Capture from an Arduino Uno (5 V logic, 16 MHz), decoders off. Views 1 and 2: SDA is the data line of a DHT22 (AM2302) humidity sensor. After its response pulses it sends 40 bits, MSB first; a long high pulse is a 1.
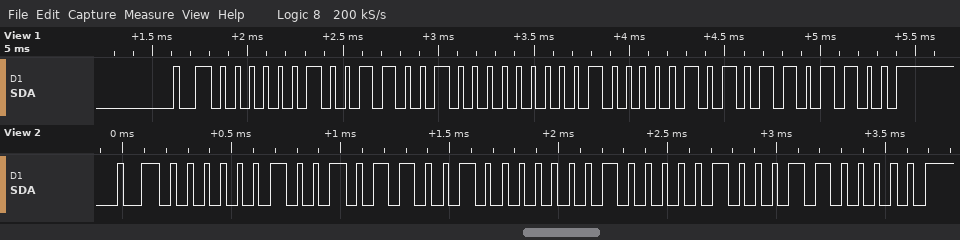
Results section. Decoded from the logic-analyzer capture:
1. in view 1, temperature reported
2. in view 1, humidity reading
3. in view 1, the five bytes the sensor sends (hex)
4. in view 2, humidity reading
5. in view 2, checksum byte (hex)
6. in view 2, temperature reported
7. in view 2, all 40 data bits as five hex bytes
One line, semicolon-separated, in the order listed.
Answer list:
26.1 °C; 61.2 %; 02 64 01 05 6C; 60.1 %; 0x60; 26.0 °C; 02 59 01 04 60
